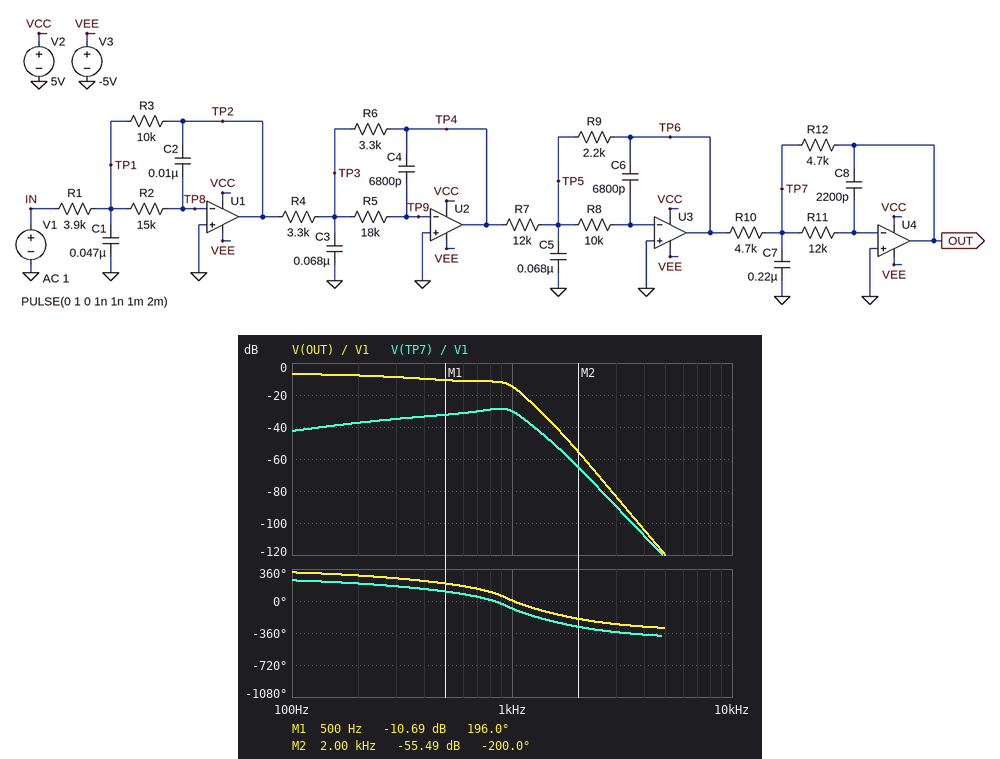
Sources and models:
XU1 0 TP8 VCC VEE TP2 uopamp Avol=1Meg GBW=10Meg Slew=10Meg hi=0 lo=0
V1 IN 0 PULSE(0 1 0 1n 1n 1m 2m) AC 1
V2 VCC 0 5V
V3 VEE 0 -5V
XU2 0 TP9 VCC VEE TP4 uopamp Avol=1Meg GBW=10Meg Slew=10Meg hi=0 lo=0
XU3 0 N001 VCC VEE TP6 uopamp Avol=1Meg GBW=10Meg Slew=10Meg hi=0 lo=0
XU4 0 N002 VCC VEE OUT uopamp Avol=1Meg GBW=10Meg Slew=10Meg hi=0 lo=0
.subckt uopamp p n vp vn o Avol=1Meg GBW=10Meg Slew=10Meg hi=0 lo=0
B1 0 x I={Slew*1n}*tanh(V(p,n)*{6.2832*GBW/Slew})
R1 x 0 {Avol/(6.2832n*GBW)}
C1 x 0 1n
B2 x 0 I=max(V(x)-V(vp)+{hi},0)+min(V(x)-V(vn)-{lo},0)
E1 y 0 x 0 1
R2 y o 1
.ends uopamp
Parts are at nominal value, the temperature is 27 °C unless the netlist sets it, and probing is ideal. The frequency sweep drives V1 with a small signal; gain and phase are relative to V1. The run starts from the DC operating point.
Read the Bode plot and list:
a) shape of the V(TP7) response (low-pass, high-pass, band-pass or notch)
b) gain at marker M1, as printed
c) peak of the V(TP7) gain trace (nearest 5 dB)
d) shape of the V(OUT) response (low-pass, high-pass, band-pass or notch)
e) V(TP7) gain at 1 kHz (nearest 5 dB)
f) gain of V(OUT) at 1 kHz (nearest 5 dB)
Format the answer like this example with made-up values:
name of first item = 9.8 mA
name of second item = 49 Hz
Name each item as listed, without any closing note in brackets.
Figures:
shape of the V(TP7) response = band-pass
gain at marker M1, as printed = -10.69 dB
peak of the V(TP7) gain trace = -30 dB
shape of the V(OUT) response = low-pass
V(TP7) gain at 1 kHz = -30 dB
gain of V(OUT) at 1 kHz = -15 dB
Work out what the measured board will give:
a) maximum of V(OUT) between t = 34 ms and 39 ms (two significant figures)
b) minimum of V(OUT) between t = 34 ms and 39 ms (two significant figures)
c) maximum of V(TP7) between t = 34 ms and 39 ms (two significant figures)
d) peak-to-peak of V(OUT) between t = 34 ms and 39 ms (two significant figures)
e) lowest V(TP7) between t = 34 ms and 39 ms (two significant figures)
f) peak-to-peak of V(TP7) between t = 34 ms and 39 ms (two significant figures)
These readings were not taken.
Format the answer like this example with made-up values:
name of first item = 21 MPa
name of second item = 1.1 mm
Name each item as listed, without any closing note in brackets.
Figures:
maximum of V(OUT) between t = 34 ms and 39 ms = 420 mV
minimum of V(OUT) between t = 34 ms and 39 ms = 52 mV
maximum of V(TP7) between t = 34 ms and 39 ms = 16 mV
peak-to-peak of V(OUT) between t = 34 ms and 39 ms = 370 mV
lowest V(TP7) between t = 34 ms and 39 ms = -16 mV
peak-to-peak of V(TP7) between t = 34 ms and 39 ms = 32 mV
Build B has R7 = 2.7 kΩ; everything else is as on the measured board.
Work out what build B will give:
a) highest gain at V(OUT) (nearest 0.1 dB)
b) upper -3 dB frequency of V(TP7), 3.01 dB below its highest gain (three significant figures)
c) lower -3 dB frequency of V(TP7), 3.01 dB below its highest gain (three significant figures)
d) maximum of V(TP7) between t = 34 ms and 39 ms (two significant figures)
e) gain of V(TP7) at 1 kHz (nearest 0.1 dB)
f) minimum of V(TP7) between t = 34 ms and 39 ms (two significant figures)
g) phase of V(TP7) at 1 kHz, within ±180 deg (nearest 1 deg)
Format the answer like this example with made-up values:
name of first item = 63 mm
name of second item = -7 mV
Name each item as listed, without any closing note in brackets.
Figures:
highest gain at V(OUT) = 6.4 dB
upper -3 dB frequency of V(TP7), 3.01 dB below its highest gain = 1.03 kHz
lower -3 dB frequency of V(TP7), 3.01 dB below its highest gain = 468 Hz
maximum of V(TP7) between t = 34 ms and 39 ms = 67 mV
gain of V(TP7) at 1 kHz = -19.1 dB
minimum of V(TP7) between t = 34 ms and 39 ms = -67 mV
phase of V(TP7) at 1 kHz, within ±180 deg = -94 deg
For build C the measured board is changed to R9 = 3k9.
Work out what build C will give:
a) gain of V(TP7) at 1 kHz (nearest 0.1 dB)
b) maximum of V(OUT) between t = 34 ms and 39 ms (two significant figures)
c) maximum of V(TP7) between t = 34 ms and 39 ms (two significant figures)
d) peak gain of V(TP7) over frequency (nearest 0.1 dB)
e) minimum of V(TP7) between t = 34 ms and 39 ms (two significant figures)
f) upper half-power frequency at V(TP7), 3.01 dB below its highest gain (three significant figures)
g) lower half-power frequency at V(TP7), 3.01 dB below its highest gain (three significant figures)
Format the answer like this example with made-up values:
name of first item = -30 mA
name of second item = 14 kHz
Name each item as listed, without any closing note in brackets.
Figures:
gain of V(TP7) at 1 kHz = -24.6 dB
maximum of V(OUT) between t = 34 ms and 39 ms = 760 mV
maximum of V(TP7) between t = 34 ms and 39 ms = 30 mV
peak gain of V(TP7) over frequency = -22.7 dB
minimum of V(TP7) between t = 34 ms and 39 ms = -30 mV
upper half-power frequency at V(TP7), 3.01 dB below its highest gain = 1.03 kHz
lower half-power frequency at V(TP7), 3.01 dB below its highest gain = 596 Hz
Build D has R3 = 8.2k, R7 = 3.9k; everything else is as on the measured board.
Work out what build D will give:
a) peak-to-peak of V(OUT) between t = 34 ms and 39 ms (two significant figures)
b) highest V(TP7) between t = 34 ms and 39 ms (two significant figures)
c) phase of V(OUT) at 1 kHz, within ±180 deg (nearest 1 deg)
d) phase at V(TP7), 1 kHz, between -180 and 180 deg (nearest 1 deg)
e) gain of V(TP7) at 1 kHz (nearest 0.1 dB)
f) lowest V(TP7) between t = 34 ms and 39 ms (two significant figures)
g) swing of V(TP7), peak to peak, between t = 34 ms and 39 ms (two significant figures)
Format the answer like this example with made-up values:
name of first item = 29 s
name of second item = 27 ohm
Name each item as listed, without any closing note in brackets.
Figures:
peak-to-peak of V(OUT) between t = 34 ms and 39 ms = 1.0 V
highest V(TP7) between t = 34 ms and 39 ms = 45 mV
phase of V(OUT) at 1 kHz, within ±180 deg = 4 deg
phase at V(TP7), 1 kHz, between -180 and 180 deg = -86 deg
gain of V(TP7) at 1 kHz = -21.8 dB
lowest V(TP7) between t = 34 ms and 39 ms = -45 mV
swing of V(TP7), peak to peak, between t = 34 ms and 39 ms = 90 mV
